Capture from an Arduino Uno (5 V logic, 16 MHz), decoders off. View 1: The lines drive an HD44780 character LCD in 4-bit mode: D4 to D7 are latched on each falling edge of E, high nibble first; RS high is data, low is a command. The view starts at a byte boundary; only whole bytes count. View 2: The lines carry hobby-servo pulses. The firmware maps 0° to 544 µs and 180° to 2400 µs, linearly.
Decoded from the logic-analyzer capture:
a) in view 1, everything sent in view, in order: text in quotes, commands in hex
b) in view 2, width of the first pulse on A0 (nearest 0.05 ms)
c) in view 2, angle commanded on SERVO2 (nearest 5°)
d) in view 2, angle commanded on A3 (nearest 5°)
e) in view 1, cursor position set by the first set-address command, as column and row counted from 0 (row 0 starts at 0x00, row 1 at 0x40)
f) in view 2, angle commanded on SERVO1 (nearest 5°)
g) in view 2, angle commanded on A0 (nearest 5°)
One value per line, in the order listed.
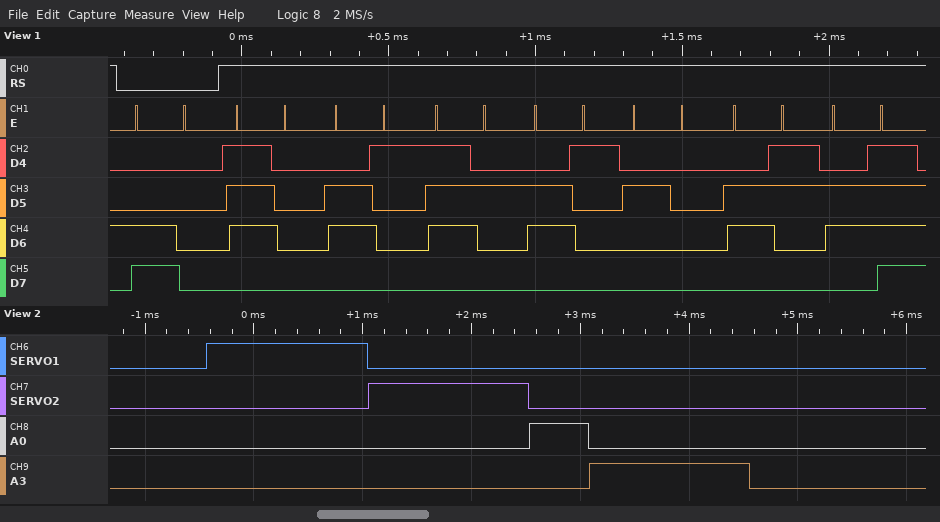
0xC0 "para co"
0.55 ms
90°
90°
column 0, row 1
90°
0°
